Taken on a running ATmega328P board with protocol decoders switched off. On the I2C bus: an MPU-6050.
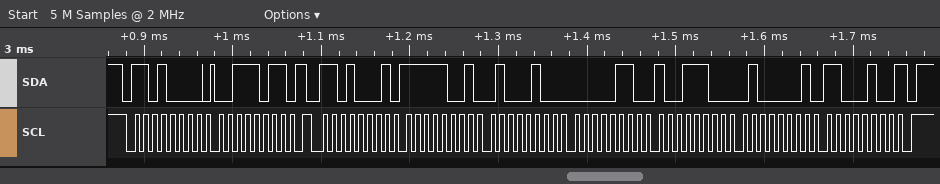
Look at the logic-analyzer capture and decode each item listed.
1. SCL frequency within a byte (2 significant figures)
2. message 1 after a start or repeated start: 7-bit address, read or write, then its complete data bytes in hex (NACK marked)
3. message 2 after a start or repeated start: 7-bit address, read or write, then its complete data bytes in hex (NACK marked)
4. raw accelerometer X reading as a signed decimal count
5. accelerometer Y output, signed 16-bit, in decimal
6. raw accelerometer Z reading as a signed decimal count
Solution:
100 kHz
0x68 write: 3B
0x68 read: F9 44 06 9C 41 C4 NACK
-1724
1692
16836
